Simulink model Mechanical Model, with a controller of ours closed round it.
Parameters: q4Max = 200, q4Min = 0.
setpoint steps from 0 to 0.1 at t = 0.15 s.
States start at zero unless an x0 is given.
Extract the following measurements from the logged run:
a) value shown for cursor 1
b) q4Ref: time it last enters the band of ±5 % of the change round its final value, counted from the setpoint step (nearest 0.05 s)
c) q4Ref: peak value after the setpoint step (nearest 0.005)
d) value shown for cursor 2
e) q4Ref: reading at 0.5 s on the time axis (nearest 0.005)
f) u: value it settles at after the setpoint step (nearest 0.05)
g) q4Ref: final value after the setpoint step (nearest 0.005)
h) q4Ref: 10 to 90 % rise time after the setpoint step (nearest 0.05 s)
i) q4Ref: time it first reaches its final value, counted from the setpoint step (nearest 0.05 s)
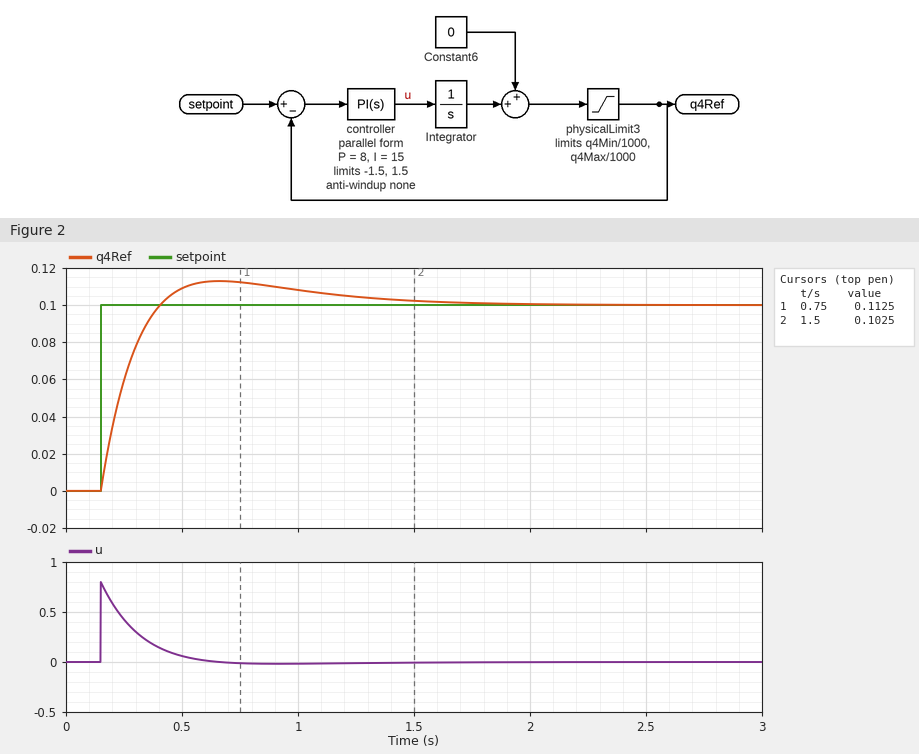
0.1125
1.05 s
0.115
0.1025
0.110
0.00
0.100
0.20 s
0.25 s
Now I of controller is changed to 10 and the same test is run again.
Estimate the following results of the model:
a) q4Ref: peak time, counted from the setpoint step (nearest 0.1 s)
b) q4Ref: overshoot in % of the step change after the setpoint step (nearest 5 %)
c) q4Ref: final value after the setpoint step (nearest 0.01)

0.6 s
10 %
0.10
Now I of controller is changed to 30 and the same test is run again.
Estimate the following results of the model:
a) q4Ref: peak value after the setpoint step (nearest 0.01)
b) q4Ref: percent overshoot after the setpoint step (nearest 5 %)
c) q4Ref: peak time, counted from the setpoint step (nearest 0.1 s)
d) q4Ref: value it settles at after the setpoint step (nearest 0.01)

0.12
20 %
0.4 s
0.10
